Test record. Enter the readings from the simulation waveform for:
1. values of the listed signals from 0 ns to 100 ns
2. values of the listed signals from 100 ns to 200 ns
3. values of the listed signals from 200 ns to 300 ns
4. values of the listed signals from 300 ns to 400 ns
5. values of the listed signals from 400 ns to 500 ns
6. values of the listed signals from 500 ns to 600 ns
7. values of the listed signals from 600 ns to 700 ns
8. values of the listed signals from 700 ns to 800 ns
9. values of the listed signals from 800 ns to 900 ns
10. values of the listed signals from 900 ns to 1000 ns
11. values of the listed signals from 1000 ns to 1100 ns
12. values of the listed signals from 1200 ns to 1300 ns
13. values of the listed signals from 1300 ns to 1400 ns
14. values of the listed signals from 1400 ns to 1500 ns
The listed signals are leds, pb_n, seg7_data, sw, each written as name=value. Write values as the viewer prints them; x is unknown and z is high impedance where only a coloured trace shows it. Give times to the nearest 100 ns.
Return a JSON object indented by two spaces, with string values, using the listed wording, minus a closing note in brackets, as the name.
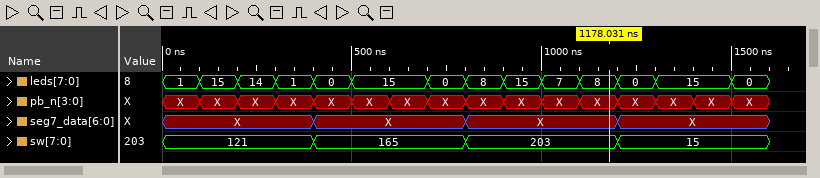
{
  "values of the listed signals from 0 ns to 100 ns": "leds=1, pb_n=X, seg7_data=X, sw=121",
  "values of the listed signals from 100 ns to 200 ns": "leds=15, pb_n=X, seg7_data=X, sw=121",
  "values of the listed signals from 200 ns to 300 ns": "leds=14, pb_n=X, seg7_data=X, sw=121",
  "values of the listed signals from 300 ns to 400 ns": "leds=1, pb_n=X, seg7_data=X, sw=121",
  "values of the listed signals from 400 ns to 500 ns": "leds=0, pb_n=X, seg7_data=X, sw=165",
  "values of the listed signals from 500 ns to 600 ns": "leds=15, pb_n=X, seg7_data=X, sw=165",
  "values of the listed signals from 600 ns to 700 ns": "leds=15, pb_n=X, seg7_data=X, sw=165",
  "values of the listed signals from 700 ns to 800 ns": "leds=0, pb_n=X, seg7_data=X, sw=165",
  "values of the listed signals from 800 ns to 900 ns": "leds=8, pb_n=X, seg7_data=X, sw=203",
  "values of the listed signals from 900 ns to 1000 ns": "leds=15, pb_n=X, seg7_data=X, sw=203",
  "values of the listed signals from 1000 ns to 1100 ns": "leds=7, pb_n=X, seg7_data=X, sw=203",
  "values of the listed signals from 1200 ns to 1300 ns": "leds=0, pb_n=X, seg7_data=X, sw=15",
  "values of the listed signals from 1300 ns to 1400 ns": "leds=15, pb_n=X, seg7_data=X, sw=15",
  "values of the listed signals from 1400 ns to 1500 ns": "leds=15, pb_n=X, seg7_data=X, sw=15"
}
